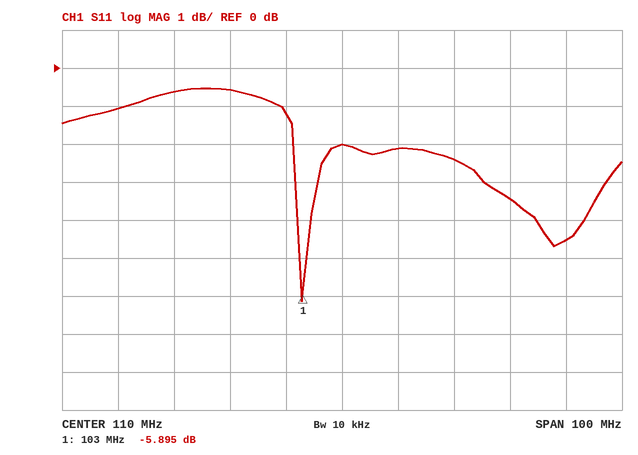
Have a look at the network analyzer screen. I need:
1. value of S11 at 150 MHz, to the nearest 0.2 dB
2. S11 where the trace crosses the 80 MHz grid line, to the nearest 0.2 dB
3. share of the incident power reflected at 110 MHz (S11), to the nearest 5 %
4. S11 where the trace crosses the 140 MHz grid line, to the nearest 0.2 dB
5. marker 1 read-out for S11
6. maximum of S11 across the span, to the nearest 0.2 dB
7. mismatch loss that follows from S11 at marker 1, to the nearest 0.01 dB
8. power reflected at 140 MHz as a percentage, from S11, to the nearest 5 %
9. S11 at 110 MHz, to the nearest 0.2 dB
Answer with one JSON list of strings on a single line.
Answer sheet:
["-4.6 dB", "-0.6 dB", "65 %", "-3.4 dB", "-5.895 dB", "-0.6 dB", "1.29 dB", "45 %", "-2.0 dB"]
